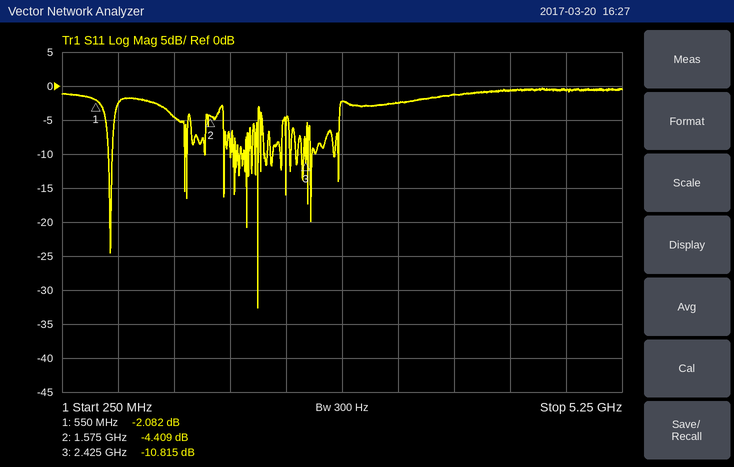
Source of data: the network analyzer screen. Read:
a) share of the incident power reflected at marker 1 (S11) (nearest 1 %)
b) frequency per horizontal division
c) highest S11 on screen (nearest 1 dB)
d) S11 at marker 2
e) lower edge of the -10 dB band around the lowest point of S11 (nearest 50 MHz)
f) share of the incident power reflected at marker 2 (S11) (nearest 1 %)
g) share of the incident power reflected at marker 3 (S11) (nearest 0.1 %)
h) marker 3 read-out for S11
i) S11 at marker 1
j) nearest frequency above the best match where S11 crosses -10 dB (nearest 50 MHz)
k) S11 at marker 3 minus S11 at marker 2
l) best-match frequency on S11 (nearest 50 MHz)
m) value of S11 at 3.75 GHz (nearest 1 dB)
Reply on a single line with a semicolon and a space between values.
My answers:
62 %; 500 MHz; 0 dB; -4.409 dB; 2.00 GHz; 36 %; 8.3 %; -10.815 dB; -2.082 dB; 2.00 GHz; -6.406 dB; 2.00 GHz; -1 dB
